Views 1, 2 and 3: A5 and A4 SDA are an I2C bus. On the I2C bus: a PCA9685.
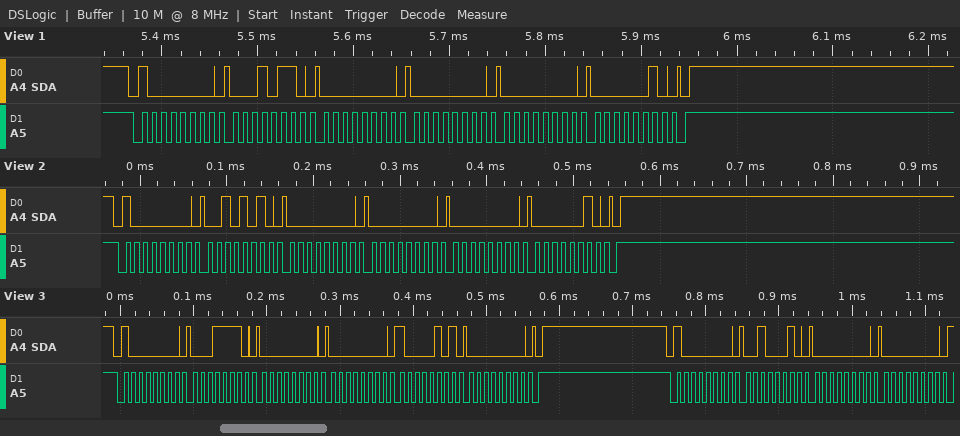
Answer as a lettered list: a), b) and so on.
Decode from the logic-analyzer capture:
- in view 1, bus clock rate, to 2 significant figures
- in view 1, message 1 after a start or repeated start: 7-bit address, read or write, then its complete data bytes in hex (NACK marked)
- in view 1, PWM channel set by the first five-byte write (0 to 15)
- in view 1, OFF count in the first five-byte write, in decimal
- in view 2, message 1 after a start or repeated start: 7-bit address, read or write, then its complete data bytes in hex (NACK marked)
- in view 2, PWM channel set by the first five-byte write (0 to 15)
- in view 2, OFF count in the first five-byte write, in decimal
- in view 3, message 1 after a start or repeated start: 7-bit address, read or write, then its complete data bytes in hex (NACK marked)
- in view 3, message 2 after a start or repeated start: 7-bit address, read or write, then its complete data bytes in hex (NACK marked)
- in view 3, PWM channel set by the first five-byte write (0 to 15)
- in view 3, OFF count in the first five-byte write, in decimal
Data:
a) 100 kHz
b) 0x40 write: 16 00 00 00 02
c) 4
d) 512
e) 0x40 write: 2A 00 00 00 02
f) 9
g) 512
h) 0x40 write: 1E 00 00 85 00
i) 0x40 write: 22 00 00
j) 6
k) 133
